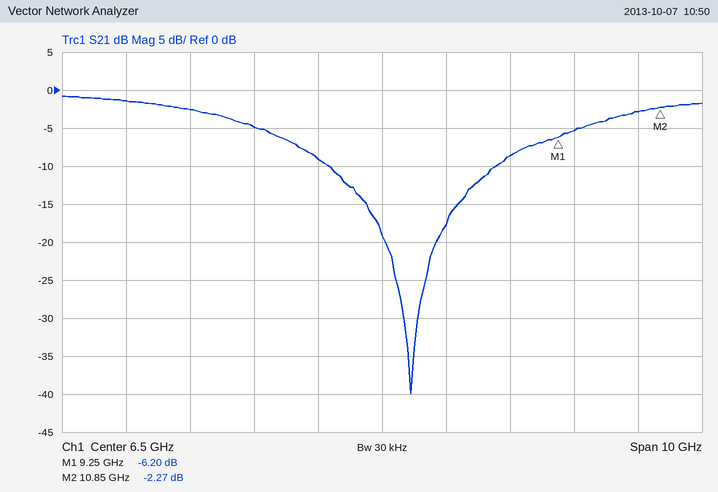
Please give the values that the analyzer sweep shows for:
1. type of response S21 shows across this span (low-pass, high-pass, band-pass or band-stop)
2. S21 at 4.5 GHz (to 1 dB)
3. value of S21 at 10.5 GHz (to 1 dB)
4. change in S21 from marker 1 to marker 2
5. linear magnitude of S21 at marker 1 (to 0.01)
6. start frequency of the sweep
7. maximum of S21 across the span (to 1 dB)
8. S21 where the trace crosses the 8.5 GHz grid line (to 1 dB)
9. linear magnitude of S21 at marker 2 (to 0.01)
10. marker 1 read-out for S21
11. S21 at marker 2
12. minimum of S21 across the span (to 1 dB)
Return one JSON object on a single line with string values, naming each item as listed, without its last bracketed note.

{"type of response S21 shows across this span": "band-stop", "S21 at 4.5 GHz": "-5 dB", "value of S21 at 10.5 GHz": "-3 dB", "change in S21 from marker 1 to marker 2": "3.93 dB", "linear magnitude of S21 at marker 1": "0.49", "start frequency of the sweep": "1.5 GHz", "maximum of S21 across the span": "-1 dB", "S21 where the trace crosses the 8.5 GHz grid line": "-9 dB", "linear magnitude of S21 at marker 2": "0.77", "marker 1 read-out for S21": "-6.20 dB", "S21 at marker 2": "-2.27 dB", "minimum of S21 across the span": "-40 dB"}
